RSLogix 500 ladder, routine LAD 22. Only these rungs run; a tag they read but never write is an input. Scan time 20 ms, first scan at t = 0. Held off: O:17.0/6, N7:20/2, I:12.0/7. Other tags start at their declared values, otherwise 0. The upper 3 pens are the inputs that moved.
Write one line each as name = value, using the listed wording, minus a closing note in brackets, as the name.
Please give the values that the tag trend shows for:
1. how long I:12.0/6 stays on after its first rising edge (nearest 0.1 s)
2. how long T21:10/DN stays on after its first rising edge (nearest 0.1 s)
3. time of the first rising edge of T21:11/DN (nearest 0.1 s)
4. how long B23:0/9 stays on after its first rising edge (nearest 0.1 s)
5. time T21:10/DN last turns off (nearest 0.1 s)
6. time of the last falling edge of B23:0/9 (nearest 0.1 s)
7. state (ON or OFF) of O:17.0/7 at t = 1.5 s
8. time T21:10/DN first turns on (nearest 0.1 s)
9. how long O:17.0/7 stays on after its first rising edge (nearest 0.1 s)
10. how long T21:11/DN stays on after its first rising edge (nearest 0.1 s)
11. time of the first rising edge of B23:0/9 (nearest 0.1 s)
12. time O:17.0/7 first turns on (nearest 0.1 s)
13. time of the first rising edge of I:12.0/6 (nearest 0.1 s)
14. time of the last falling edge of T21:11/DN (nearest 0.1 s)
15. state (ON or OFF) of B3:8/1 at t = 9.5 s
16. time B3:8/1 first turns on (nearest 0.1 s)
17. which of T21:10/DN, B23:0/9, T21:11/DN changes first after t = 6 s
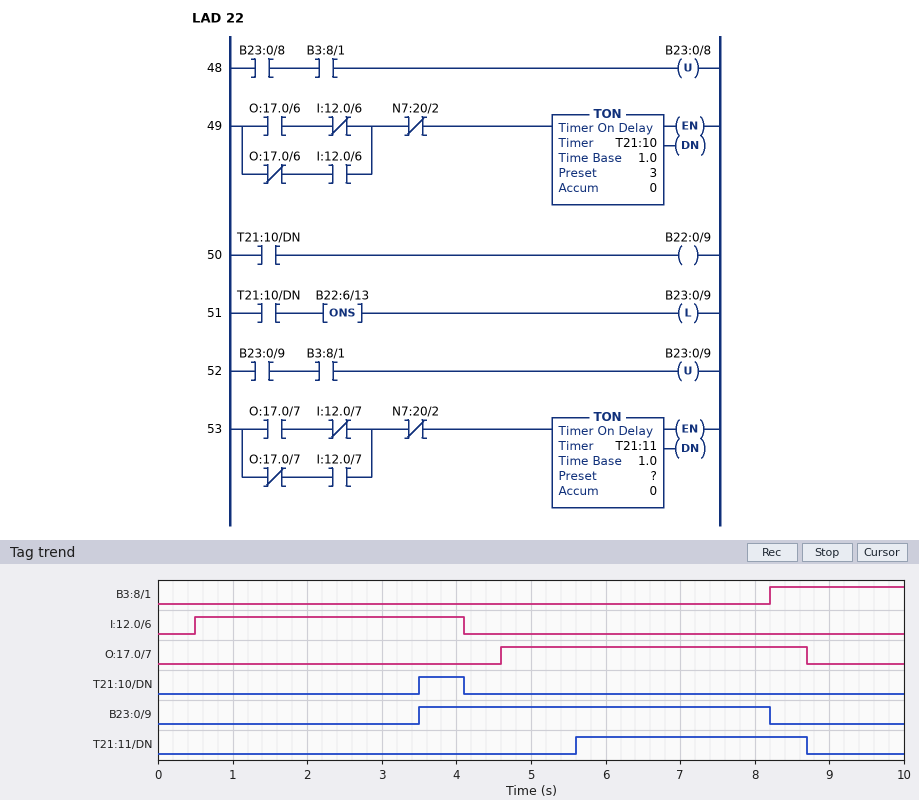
how long I:12.0/6 stays on after its first rising edge = 3.6 s
how long T21:10/DN stays on after its first rising edge = 0.6 s
time of the first rising edge of T21:11/DN = 5.6 s
how long B23:0/9 stays on after its first rising edge = 4.7 s
time T21:10/DN last turns off = 4.1 s
time of the last falling edge of B23:0/9 = 8.2 s
state (ON or OFF) of O:17.0/7 at t = 1.5 s = OFF
time T21:10/DN first turns on = 3.5 s
how long O:17.0/7 stays on after its first rising edge = 4.1 s
how long T21:11/DN stays on after its first rising edge = 3.1 s
time of the first rising edge of B23:0/9 = 3.5 s
time O:17.0/7 first turns on = 4.6 s
time of the first rising edge of I:12.0/6 = 0.5 s
time of the last falling edge of T21:11/DN = 8.7 s
state (ON or OFF) of B3:8/1 at t = 9.5 s = ON
time B3:8/1 first turns on = 8.2 s
which of T21:10/DN, B23:0/9, T21:11/DN changes first after t = 6 s = B23:0/9
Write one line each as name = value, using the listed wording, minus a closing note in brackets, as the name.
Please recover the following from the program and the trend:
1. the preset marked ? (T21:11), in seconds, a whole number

the preset marked ? (T21:11), in seconds, a whole number = 1 s
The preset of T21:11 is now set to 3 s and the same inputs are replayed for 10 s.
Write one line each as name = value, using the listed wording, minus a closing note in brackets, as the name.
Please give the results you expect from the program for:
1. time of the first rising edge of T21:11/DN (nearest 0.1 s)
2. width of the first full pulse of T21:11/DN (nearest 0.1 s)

time of the first rising edge of T21:11/DN = 7.6 s
width of the first full pulse of T21:11/DN = 1.1 s
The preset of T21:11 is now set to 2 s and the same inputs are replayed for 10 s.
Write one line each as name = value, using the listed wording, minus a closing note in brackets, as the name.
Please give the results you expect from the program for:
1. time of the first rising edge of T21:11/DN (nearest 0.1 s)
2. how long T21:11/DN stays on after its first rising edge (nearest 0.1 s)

time of the first rising edge of T21:11/DN = 6.6 s
how long T21:11/DN stays on after its first rising edge = 2.1 s
